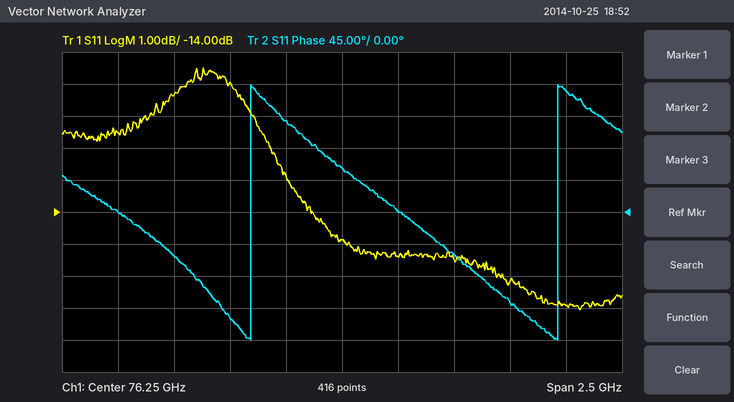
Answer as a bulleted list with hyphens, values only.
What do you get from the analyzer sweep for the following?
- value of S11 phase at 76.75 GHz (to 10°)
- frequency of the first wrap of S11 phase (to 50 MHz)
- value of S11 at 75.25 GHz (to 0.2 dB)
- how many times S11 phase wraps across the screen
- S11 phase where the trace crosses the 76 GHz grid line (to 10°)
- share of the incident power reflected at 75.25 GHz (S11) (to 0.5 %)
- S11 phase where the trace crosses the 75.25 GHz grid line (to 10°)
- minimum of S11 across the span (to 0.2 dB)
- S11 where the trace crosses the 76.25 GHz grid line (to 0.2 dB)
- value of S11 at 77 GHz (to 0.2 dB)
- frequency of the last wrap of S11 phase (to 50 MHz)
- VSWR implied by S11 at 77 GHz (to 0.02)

- -60°
- 75.85 GHz
- -11.6 dB
- 2
- 130°
- 7.0 %
- 0°
- -17.0 dB
- -14.8 dB
- -16.2 dB
- 77.20 GHz
- 1.36
